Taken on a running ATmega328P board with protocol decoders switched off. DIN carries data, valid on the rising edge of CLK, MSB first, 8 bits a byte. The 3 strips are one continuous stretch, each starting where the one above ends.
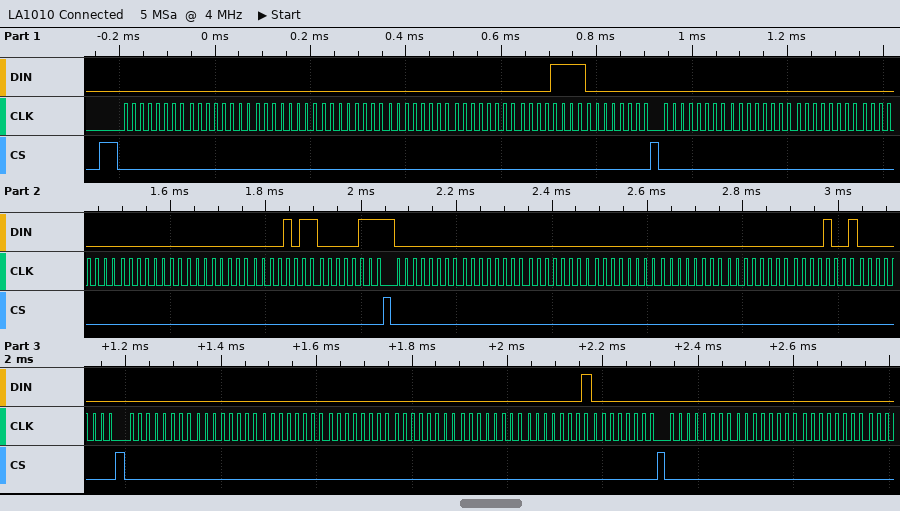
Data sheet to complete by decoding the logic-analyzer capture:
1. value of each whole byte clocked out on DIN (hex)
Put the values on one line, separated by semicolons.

0x00 0x00 0x00 0x00 0x00 0x00 0x0F 0x00 0x00 0x00 0x00 0x00 0x00 0x00 0x0B 0x07 0x00 0x00 0x00 0x00 0x00 0x00 0x09 0x00 0x00 0x00 0x00 0x00 0x00 0x00 0x01 0x00 0x00 0x00 0x00
